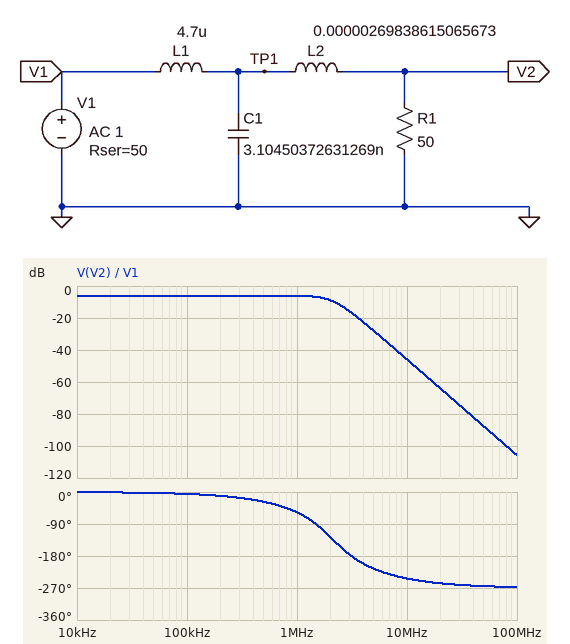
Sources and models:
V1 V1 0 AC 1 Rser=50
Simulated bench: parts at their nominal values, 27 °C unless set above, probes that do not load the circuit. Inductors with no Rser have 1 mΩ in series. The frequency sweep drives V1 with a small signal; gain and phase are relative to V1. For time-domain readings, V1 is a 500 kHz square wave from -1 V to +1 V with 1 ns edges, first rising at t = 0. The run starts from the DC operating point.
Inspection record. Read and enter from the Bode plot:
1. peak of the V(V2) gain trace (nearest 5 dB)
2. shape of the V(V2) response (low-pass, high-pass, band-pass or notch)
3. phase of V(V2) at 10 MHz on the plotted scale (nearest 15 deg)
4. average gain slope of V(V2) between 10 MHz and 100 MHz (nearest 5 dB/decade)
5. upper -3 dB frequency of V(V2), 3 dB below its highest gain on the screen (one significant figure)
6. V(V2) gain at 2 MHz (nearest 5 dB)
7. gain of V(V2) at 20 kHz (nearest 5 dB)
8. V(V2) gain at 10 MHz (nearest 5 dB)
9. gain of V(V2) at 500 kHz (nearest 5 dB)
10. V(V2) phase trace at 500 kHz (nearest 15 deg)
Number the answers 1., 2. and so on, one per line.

1. -5 dB
2. low-pass
3. -240 deg
4. -60 dB/decade
5. 2 MHz
6. -10 dB
7. -5 dB
8. -45 dB
9. -5 dB
10. -30 deg
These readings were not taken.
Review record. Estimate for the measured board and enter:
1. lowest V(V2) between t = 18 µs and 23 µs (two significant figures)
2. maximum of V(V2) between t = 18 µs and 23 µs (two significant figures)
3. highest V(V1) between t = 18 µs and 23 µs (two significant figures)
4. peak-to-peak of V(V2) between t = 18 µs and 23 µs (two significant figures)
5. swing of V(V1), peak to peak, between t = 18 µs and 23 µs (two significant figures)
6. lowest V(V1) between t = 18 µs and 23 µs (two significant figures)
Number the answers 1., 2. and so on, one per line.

1. -570 mV
2. 570 mV
3. 1.5 V
4. 1.1 V
5. 3.0 V
6. -1.5 V
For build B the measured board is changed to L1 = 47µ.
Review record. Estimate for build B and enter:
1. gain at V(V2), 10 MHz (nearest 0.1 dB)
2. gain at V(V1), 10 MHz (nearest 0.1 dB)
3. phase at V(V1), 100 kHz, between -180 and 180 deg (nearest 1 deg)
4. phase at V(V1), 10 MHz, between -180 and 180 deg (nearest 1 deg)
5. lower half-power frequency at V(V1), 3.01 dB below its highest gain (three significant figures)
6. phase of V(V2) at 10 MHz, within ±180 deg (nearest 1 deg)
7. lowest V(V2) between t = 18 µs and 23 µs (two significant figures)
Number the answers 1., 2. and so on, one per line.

1. -65.9 dB
2. 0 dB
3. 13 deg
4. 1 deg
5. 268 kHz
6. 108 deg
7. -390 mV
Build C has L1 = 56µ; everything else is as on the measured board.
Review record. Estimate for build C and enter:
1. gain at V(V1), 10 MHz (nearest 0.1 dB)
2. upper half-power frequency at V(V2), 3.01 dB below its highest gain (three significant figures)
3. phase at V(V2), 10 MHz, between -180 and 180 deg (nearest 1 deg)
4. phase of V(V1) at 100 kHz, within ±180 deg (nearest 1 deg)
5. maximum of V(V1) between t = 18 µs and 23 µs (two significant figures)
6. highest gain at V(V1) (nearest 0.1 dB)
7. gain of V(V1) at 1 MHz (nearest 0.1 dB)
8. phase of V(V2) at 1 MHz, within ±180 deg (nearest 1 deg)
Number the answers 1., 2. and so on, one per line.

1. 0 dB
2. 308 kHz
3. 108 deg
4. 15 deg
5. 1.4 V
6. 0 dB
7. -0.2 dB
8. -131 deg
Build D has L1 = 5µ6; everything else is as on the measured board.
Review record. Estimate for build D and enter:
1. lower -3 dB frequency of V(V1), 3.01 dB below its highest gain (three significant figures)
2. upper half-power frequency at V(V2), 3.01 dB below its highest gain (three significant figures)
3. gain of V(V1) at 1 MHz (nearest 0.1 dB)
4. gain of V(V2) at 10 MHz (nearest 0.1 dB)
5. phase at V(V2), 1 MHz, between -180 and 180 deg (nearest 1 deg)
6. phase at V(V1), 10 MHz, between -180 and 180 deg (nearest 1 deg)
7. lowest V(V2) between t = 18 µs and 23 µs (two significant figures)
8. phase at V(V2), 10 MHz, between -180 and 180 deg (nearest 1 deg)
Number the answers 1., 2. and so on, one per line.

1. 2.34 MHz
2. 1.92 MHz
3. -7.4 dB
4. -47.4 dB
5. -61 deg
6. 8 deg
7. -570 mV
8. 115 deg
